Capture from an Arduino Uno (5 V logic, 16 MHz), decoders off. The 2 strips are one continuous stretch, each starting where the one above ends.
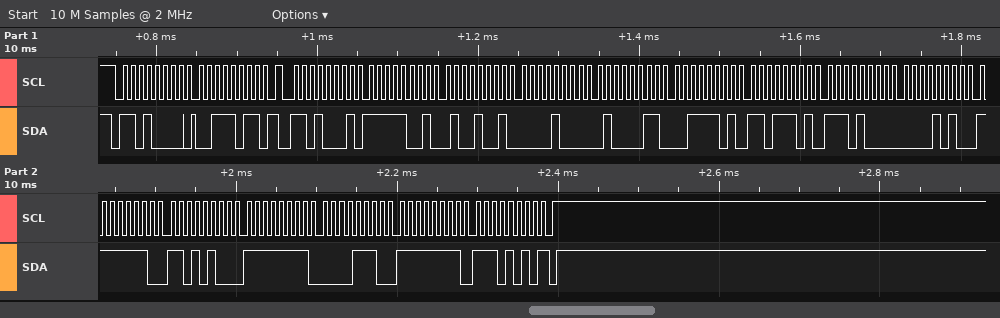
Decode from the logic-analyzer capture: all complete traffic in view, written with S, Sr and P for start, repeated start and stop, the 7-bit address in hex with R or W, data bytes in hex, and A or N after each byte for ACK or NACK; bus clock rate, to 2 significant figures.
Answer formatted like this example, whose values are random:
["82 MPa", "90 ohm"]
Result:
["S 68W A 3B A Sr 68R A F9 A 49 A 08 A 43 A 3D A DD A E8 A 0A A FE A D4 A FF A 0E A FF A EA N P", "100 kHz"]
